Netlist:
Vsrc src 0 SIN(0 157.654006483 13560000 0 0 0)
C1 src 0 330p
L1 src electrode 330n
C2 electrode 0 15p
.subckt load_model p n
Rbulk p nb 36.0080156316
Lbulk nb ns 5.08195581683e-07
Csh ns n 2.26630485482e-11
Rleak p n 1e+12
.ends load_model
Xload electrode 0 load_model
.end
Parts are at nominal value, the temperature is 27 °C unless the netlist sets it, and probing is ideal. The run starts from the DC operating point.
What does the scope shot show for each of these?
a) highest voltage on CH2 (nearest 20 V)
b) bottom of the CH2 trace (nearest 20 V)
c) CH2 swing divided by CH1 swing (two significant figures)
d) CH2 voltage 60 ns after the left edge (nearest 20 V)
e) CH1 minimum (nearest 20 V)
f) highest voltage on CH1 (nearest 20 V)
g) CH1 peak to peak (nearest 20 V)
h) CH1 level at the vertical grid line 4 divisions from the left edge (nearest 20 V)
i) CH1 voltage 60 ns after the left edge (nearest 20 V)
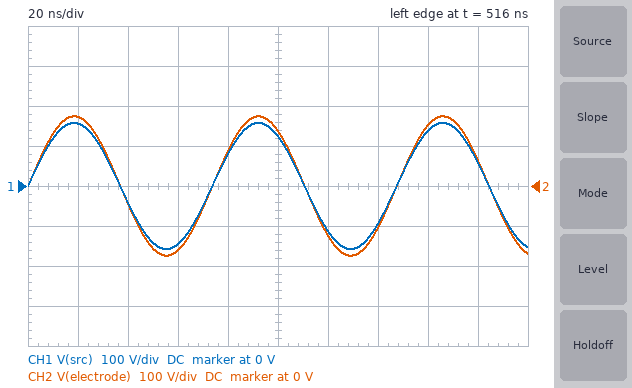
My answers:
180 V
-180 V
1.1
-160 V
-160 V
160 V
320 V
80 V
-140 V
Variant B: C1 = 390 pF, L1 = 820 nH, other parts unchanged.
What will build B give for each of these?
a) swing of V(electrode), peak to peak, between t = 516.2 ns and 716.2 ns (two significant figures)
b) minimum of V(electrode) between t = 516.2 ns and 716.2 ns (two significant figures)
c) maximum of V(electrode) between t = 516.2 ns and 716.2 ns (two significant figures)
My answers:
410 V
-210 V
210 V
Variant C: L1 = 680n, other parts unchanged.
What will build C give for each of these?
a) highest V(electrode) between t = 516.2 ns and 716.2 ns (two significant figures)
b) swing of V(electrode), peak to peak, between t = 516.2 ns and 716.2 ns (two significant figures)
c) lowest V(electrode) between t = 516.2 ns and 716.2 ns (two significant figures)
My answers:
200 V
390 V
-200 V
